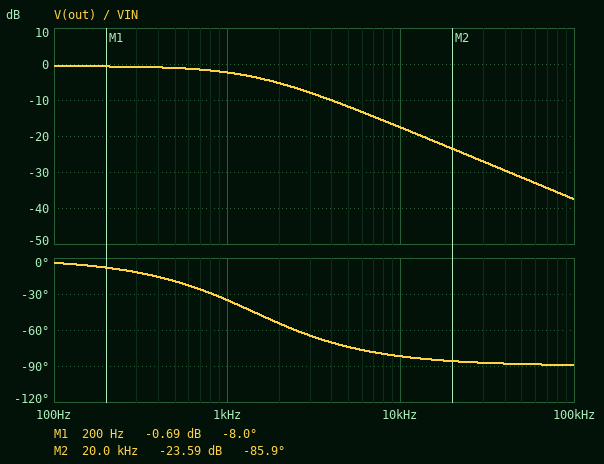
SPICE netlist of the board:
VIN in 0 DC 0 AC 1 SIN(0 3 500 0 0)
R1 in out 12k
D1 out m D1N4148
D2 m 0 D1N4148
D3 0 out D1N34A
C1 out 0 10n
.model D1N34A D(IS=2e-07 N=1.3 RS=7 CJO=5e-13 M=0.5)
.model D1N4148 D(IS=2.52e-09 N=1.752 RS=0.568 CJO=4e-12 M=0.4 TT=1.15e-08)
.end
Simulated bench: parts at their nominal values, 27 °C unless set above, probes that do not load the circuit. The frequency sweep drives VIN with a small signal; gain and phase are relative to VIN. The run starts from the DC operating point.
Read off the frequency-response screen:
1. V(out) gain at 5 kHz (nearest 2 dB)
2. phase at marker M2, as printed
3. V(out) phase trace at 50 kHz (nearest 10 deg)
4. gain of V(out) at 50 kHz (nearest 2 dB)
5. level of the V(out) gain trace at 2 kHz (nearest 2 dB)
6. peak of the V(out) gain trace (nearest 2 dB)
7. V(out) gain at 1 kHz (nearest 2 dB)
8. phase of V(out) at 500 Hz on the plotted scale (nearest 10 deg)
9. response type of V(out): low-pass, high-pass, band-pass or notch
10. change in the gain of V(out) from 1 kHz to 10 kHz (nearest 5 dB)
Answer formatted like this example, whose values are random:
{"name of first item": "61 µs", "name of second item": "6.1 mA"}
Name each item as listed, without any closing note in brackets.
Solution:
{"V(out) gain at 5 kHz": "-12 dB", "phase at marker M2, as printed": "-85.9 deg", "V(out) phase trace at 50 kHz": "-90 deg", "gain of V(out) at 50 kHz": "-32 dB", "level of the V(out) gain trace at 2 kHz": "-6 dB", "peak of the V(out) gain trace": "0 dB", "V(out) gain at 1 kHz": "-2 dB", "phase of V(out) at 500 Hz on the plotted scale": "-20 deg", "response type of V(out): low-pass, high-pass, band-pass or notch": "low-pass", "change in the gain of V(out) from 1 kHz to 10 kHz": "-15 dB"}
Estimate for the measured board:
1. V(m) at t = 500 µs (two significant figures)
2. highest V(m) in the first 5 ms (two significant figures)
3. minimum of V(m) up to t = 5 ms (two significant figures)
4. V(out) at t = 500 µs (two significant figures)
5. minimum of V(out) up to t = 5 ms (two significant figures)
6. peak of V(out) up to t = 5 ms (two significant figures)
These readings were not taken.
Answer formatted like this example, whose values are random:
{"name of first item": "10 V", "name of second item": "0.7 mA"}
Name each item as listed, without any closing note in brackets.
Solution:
{"V(m) at t = 500 µs": "500 mV", "highest V(m) in the first 5 ms": "500 mV", "minimum of V(m) up to t = 5 ms": "-120 mV", "V(out) at t = 500 µs": "1.0 V", "minimum of V(out) up to t = 5 ms": "-240 mV", "peak of V(out) up to t = 5 ms": "1.0 V"}
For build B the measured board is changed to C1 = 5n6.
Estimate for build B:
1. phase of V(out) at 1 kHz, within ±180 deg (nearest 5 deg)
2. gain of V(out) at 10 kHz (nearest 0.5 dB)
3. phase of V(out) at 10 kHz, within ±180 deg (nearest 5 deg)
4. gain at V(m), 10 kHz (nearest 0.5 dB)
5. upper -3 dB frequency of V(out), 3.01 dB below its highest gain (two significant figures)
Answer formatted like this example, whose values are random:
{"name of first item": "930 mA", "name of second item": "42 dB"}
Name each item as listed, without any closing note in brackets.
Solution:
{"phase of V(out) at 1 kHz, within ±180 deg": "-20 deg", "gain of V(out) at 10 kHz": "-13.0 dB", "phase of V(out) at 10 kHz, within ±180 deg": "-75 deg", "gain at V(m), 10 kHz": "-19.0 dB", "upper -3 dB frequency of V(out), 3.01 dB below its highest gain": "2.5 kHz"}
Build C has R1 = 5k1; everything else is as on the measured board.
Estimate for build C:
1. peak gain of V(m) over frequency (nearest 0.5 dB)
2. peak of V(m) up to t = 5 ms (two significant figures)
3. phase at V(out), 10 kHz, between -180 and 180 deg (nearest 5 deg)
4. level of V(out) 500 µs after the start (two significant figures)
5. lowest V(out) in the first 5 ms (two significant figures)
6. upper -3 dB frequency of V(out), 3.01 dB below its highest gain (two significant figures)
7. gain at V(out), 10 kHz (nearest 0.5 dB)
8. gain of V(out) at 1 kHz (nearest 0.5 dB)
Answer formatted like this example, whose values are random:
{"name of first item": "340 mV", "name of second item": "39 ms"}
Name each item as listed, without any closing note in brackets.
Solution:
{"peak gain of V(m) over frequency": "-6.5 dB", "peak of V(m) up to t = 5 ms": "540 mV", "phase at V(out), 10 kHz, between -180 and 180 deg": "-70 deg", "level of V(out) 500 µs after the start": "1.1 V", "lowest V(out) in the first 5 ms": "-270 mV", "upper -3 dB frequency of V(out), 3.01 dB below its highest gain": "3.2 kHz", "gain at V(out), 10 kHz": "-10.5 dB", "gain of V(out) at 1 kHz": "-0.5 dB"}
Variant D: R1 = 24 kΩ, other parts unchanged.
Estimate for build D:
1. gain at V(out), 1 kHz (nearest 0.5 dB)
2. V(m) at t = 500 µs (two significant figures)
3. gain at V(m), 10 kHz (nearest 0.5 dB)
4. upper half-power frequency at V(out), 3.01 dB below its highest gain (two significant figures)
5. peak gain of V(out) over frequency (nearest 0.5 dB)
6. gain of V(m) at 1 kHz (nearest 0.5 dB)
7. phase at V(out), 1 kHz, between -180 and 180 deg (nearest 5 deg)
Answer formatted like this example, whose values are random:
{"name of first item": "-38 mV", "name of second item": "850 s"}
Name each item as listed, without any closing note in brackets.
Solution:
{"gain at V(out), 1 kHz": "-5.5 dB", "V(m) at t = 500 µs": "470 mV", "gain at V(m), 10 kHz": "-29.5 dB", "upper half-power frequency at V(out), 3.01 dB below its highest gain": "760 Hz", "peak gain of V(out) over frequency": "-1.0 dB", "gain of V(m) at 1 kHz": "-11.5 dB", "phase at V(out), 1 kHz, between -180 and 180 deg": "-55 deg"}
